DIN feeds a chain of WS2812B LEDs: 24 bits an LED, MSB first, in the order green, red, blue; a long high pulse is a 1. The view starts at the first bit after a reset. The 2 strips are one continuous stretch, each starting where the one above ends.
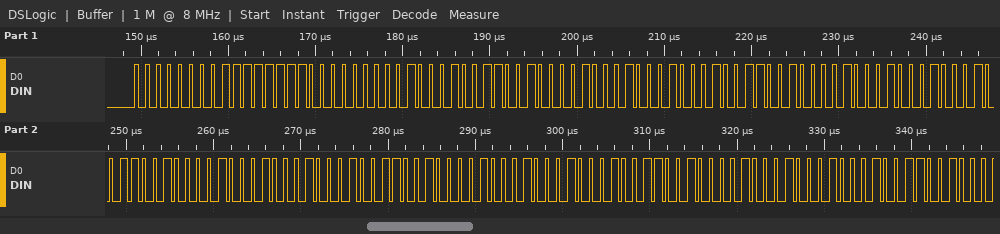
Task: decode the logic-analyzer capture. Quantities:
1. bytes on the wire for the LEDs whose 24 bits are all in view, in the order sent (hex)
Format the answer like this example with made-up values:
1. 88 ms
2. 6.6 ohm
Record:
1. 00 FF 00 44 C8 44 44 C8 44 44 C8 44 44 C8 44 44 C8 44
